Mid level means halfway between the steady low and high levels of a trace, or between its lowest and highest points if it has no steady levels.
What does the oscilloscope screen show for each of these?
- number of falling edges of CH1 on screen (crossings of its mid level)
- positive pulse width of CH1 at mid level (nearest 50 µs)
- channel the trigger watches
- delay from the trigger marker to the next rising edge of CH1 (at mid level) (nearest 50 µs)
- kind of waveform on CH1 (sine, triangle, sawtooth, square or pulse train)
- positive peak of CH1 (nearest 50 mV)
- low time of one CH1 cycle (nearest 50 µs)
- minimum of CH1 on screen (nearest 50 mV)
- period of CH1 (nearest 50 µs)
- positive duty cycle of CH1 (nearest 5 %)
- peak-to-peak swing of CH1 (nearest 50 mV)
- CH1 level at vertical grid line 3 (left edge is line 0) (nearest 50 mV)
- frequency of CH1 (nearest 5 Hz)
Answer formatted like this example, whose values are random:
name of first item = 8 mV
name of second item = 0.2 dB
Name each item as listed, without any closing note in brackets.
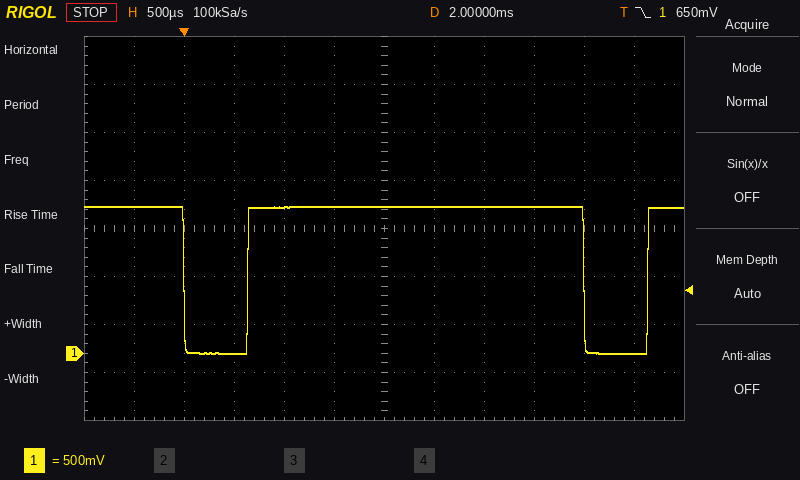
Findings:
number of falling edges of CH1 on screen = 2
positive pulse width of CH1 at mid level = 3.35 ms
channel the trigger watches = CH1
delay from the trigger marker to the next rising edge of CH1 (at mid level) = 650 µs
kind of waveform on CH1 = pulse train
positive peak of CH1 = 1.55 V
low time of one CH1 cycle = 650 µs
minimum of CH1 on screen = 0 mV
period of CH1 = 4.00 ms
positive duty cycle of CH1 = 85 %
peak-to-peak swing of CH1 = 1.55 V
CH1 level at vertical grid line 3 (left edge is line 0) = 0 mV
frequency of CH1 = 250 Hz
